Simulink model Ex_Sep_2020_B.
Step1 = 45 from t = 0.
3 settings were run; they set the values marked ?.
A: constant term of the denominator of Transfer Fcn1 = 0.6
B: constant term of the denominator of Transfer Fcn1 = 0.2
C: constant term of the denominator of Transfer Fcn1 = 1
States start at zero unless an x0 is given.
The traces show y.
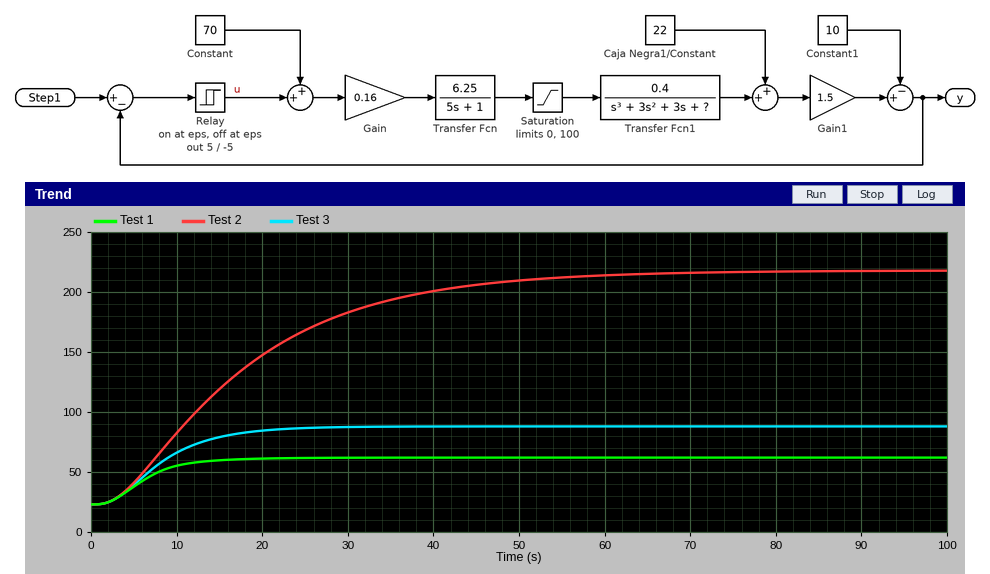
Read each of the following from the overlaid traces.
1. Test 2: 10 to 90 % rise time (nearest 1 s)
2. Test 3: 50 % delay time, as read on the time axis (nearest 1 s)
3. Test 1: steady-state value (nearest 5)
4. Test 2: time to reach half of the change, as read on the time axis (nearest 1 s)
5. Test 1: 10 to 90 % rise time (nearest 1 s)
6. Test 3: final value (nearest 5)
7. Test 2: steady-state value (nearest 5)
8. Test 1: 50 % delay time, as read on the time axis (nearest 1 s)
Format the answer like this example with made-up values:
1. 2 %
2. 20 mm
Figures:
1. 33 s
2. 8 s
3. 60
4. 15 s
5. 10 s
6. 90
7. 220
8. 6 s
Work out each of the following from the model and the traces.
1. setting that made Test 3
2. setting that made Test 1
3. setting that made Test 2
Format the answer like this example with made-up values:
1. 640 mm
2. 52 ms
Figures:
1. A
2. C
3. B
